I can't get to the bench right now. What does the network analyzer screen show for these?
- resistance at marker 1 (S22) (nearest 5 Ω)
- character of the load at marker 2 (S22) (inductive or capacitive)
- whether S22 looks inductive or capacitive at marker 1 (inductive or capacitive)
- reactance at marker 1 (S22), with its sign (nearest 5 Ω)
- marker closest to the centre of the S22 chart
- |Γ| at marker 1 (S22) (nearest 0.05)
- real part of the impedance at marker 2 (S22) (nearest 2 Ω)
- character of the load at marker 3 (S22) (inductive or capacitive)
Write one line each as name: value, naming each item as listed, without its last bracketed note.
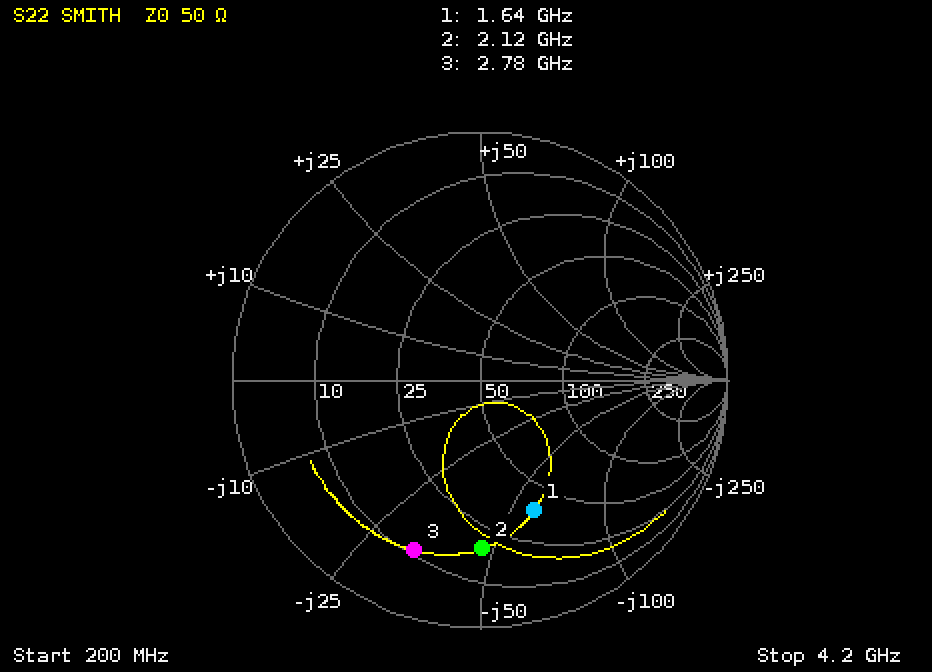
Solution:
resistance at marker 1 (S22): 40 Ω
character of the load at marker 2 (S22): capacitive
whether S22 looks inductive or capacitive at marker 1: capacitive
reactance at marker 1 (S22), with its sign: -60 Ω
marker closest to the centre of the S22 chart: marker 1
|Γ| at marker 1 (S22): 0.55
real part of the impedance at marker 2 (S22): 18 Ω
character of the load at marker 3 (S22): capacitive
